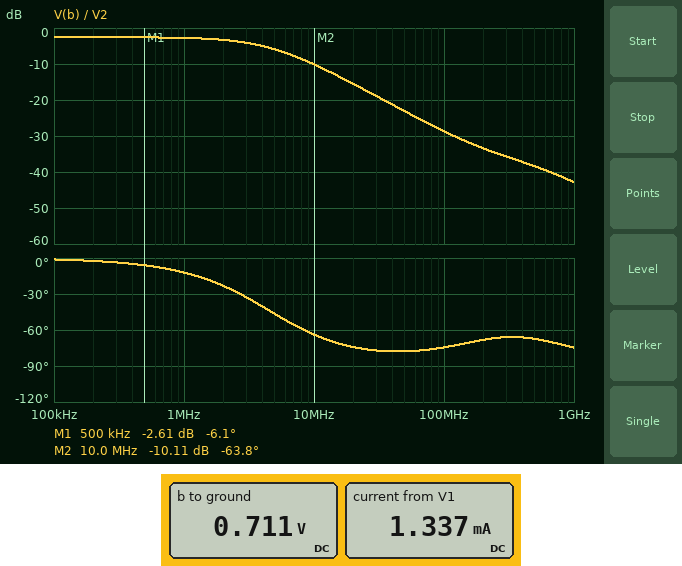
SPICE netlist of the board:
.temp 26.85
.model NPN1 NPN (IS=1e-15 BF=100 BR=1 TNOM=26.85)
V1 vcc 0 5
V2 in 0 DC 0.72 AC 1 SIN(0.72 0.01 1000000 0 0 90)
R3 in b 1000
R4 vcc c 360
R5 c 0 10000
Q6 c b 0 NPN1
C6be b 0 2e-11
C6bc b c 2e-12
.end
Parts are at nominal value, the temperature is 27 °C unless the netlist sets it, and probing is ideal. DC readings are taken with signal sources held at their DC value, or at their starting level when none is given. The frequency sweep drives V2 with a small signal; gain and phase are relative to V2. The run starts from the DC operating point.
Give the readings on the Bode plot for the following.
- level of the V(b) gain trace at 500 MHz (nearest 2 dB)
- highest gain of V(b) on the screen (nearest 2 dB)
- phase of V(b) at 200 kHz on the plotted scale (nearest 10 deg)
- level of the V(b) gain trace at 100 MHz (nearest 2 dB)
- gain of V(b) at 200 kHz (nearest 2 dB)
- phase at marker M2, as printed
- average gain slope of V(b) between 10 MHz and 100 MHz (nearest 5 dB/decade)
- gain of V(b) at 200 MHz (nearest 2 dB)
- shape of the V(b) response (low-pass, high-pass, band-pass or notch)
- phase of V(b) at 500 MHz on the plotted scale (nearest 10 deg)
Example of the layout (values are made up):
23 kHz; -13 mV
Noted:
-38 dB; -2 dB; 0 deg; -28 dB; -2 dB; -63.8 deg; -20 dB/decade; -34 dB; low-pass; -70 deg
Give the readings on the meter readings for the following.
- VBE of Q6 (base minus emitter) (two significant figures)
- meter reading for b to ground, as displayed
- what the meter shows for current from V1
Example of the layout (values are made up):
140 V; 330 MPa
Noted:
710 mV; 0.711 V; 1.337 mA
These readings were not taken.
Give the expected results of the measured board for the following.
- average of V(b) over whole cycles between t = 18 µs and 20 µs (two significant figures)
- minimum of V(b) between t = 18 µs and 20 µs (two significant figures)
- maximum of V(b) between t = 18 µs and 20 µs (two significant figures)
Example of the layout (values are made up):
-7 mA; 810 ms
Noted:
710 mV; 700 mV; 720 mV
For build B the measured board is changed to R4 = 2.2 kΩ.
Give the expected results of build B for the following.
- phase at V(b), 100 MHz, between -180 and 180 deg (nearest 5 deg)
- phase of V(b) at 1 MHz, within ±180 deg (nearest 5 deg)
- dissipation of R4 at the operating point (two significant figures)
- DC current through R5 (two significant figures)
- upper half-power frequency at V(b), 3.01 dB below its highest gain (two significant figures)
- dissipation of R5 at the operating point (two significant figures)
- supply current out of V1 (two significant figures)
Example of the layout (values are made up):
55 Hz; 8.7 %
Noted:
-40 deg; -35 deg; 2.8 mW; 250 µA; 1.4 MHz; 630 µW; 1.1 mA
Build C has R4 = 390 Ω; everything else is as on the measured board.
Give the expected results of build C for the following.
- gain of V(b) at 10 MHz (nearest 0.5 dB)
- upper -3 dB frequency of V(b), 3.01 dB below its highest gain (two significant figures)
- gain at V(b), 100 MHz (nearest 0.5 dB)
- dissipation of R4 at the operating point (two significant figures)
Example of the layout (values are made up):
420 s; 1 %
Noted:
-10.5 dB; 4.4 MHz; -29.0 dB; 690 µW
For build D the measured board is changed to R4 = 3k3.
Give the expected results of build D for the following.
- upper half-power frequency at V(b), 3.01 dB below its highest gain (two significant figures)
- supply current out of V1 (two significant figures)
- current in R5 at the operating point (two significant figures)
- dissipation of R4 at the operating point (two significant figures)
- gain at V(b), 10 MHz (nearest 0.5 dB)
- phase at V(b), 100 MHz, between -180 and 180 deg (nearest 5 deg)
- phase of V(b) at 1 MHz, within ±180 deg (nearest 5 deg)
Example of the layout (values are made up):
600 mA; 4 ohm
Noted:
1.1 MHz; 1.0 mA; 160 µA; 3.6 mW; -21.5 dB; -35 deg; -40 deg
